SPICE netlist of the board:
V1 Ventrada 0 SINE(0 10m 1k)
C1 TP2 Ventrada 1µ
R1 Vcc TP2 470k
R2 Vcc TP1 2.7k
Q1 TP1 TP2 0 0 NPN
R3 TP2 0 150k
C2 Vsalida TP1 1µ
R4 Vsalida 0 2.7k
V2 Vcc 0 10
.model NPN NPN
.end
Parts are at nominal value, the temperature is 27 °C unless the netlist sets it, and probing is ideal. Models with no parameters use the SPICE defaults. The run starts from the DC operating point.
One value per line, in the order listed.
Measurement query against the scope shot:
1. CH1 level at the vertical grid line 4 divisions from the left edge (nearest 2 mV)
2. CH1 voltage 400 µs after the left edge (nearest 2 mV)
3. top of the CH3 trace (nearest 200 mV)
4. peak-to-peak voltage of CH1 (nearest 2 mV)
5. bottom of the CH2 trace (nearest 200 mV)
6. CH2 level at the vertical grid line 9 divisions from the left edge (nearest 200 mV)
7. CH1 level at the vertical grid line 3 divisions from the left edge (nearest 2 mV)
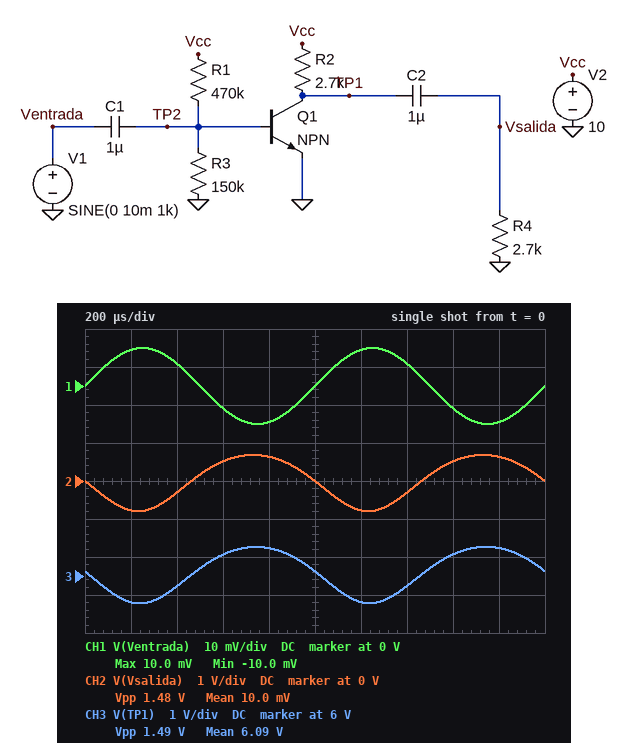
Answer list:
-10 mV
6 mV
6.8 V
20 mV
-800 mV
600 mV
-6 mV
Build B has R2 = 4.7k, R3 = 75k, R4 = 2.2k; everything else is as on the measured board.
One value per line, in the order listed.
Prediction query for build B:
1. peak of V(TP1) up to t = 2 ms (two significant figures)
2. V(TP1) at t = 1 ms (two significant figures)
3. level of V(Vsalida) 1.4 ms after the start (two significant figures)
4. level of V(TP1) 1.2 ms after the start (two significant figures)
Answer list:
6.1 V
5.6 V
-250 mV
5.0 V
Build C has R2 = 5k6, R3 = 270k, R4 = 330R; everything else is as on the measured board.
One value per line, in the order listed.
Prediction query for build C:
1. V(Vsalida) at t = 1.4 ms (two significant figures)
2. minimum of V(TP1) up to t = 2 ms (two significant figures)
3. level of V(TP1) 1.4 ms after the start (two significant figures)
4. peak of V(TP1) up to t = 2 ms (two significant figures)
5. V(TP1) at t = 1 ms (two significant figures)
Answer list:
-78 mV
340 mV
420 mV
800 mV
670 mV
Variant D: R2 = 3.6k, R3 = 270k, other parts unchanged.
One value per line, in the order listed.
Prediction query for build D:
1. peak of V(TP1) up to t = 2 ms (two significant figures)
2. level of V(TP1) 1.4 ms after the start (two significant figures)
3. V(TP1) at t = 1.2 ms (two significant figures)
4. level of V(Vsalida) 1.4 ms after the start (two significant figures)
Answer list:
4.9 V
3.5 V
2.9 V
-390 mV
